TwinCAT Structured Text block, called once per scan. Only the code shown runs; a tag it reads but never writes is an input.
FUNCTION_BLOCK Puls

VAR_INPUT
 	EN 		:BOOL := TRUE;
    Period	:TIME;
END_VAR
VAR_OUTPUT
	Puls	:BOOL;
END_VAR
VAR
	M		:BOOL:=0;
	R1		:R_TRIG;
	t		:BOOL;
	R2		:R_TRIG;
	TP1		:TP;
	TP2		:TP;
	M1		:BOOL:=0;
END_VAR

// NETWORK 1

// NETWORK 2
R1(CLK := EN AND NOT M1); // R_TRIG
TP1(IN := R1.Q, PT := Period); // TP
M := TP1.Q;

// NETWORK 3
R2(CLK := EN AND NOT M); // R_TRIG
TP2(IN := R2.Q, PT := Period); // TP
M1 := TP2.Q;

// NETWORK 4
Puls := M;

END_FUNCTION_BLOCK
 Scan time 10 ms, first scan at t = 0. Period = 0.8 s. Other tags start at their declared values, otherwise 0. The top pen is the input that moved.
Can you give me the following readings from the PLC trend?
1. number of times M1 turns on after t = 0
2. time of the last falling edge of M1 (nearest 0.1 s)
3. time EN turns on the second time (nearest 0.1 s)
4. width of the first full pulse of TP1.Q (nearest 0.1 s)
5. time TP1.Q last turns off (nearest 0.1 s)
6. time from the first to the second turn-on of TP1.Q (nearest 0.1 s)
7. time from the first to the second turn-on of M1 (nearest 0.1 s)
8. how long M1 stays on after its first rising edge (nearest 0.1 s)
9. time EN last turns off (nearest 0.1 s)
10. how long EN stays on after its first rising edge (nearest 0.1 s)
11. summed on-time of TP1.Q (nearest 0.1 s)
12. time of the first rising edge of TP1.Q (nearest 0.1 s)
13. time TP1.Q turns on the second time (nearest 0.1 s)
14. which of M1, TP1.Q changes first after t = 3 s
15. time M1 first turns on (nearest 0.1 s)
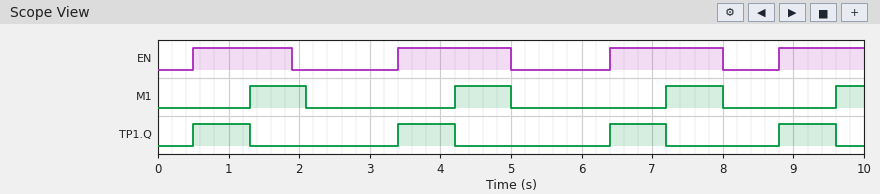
4
8.0 s
3.4 s
0.8 s
9.6 s
2.9 s
2.9 s
0.8 s
8.0 s
1.4 s
3.2 s
0.5 s
3.4 s
TP1.Q
1.3 s
